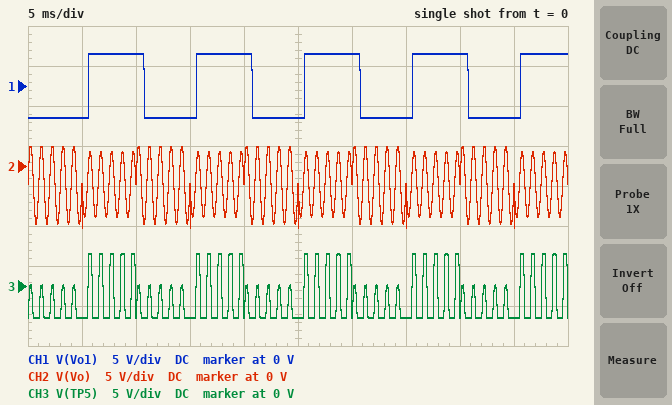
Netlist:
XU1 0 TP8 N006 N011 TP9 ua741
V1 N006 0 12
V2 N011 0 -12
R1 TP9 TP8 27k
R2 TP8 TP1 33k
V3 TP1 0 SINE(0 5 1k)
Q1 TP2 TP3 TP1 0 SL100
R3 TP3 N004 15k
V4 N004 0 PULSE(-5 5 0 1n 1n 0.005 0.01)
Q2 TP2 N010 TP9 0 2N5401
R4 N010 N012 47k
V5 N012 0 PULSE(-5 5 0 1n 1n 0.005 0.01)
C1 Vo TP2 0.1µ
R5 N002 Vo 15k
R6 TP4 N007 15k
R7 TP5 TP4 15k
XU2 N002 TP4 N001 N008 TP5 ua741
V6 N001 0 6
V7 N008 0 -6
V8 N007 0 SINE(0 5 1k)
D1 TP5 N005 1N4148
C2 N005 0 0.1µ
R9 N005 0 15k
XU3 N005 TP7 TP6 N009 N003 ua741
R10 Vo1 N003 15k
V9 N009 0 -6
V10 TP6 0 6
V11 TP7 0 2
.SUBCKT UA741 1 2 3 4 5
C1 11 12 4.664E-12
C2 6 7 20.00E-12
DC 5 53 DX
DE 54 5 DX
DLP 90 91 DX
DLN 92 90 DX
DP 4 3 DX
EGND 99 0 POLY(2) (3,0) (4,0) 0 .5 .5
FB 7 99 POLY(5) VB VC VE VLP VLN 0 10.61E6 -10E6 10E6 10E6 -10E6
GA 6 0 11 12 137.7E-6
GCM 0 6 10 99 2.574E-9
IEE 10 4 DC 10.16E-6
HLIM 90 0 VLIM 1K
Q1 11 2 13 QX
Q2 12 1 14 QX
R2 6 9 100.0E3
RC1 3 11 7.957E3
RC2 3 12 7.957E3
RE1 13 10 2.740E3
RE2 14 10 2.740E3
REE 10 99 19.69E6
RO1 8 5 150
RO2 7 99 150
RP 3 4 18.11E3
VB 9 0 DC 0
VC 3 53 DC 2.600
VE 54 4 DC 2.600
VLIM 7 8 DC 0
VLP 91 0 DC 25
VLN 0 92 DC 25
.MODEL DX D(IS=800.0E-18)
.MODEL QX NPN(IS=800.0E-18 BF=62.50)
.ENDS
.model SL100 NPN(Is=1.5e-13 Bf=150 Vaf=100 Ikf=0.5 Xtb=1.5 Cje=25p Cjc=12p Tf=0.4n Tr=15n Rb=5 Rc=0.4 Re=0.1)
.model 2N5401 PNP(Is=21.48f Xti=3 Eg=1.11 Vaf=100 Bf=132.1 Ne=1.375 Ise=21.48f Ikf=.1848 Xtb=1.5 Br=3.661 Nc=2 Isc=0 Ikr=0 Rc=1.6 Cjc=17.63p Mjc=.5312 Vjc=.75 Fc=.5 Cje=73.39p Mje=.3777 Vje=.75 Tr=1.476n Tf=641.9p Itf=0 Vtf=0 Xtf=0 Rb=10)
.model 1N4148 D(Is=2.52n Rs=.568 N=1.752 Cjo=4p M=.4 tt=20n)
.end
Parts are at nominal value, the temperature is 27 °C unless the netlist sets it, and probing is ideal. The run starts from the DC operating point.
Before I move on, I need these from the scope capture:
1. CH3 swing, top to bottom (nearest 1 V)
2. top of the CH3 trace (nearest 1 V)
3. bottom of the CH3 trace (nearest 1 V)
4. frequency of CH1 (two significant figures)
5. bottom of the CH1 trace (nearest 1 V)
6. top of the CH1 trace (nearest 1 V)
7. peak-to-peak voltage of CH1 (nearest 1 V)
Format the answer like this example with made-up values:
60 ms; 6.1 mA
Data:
8 V; 4 V; -4 V; 100 Hz; -4 V; 4 V; 8 V
